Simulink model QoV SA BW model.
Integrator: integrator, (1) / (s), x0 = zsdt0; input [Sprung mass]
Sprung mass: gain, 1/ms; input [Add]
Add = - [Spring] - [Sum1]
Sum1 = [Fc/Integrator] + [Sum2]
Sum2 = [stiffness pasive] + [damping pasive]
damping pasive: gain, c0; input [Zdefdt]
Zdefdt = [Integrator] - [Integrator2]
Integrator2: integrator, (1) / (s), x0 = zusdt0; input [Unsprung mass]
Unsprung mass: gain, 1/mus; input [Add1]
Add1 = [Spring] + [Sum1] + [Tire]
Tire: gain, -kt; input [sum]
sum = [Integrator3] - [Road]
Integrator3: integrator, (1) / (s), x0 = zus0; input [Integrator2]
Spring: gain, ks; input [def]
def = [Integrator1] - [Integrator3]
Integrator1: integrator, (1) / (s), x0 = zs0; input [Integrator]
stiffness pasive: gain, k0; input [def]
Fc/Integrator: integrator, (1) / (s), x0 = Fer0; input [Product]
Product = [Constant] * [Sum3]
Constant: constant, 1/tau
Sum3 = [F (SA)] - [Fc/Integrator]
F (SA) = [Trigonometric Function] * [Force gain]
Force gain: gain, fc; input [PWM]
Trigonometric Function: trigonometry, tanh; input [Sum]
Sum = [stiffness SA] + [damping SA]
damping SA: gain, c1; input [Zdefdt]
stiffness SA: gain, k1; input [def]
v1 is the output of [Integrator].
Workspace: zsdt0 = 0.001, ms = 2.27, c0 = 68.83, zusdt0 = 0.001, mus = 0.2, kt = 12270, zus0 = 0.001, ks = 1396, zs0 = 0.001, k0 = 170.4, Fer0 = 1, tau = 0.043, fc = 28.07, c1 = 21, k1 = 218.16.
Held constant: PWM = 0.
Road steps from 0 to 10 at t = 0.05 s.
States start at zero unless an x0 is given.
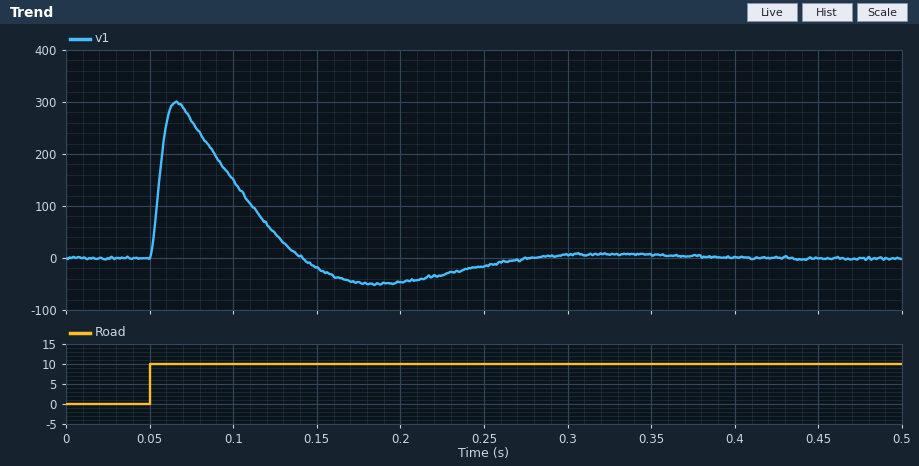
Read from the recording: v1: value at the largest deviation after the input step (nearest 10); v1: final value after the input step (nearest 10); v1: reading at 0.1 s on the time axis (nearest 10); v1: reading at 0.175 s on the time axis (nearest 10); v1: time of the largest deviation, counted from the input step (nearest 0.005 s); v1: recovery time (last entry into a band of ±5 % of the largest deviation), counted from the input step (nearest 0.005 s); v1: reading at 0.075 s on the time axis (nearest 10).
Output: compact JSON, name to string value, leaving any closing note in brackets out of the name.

{"v1: value at the largest deviation after the input step": "300", "v1: final value after the input step": "0", "v1: reading at 0.1 s on the time axis": "150", "v1: reading at 0.175 s on the time axis": "-50", "v1: time of the largest deviation, counted from the input step": "0.015 s", "v1: recovery time (last entry into a band of ±5 % of the largest deviation), counted from the input step": "0.200 s", "v1: reading at 0.075 s on the time axis": "260"}
